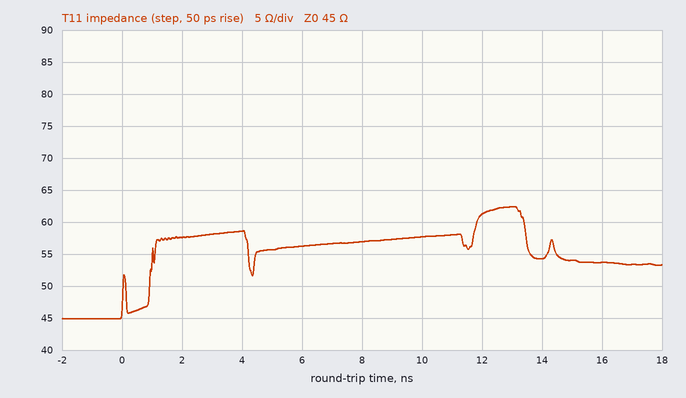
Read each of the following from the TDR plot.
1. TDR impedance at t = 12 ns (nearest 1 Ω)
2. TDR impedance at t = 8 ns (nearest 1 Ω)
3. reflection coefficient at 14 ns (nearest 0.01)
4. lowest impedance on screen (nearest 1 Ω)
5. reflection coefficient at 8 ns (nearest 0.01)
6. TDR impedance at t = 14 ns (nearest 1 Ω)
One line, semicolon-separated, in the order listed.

61 Ω; 57 Ω; +0.09; 45 Ω; +0.12; 54 Ω
